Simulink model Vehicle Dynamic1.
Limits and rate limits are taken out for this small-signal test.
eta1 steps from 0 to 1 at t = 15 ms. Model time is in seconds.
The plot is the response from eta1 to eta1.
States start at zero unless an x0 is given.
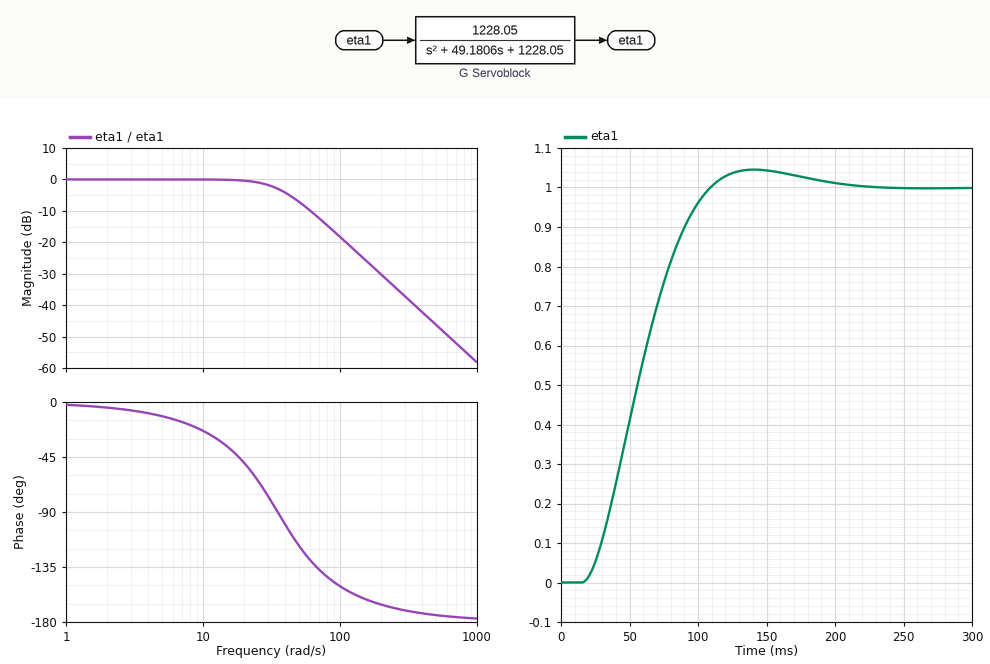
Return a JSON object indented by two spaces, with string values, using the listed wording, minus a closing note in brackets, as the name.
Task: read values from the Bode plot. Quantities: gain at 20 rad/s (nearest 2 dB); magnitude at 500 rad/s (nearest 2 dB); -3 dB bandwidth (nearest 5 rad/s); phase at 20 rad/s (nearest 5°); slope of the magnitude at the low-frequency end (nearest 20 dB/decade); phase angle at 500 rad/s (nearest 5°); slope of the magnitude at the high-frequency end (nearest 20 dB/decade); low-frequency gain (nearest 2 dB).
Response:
{
  "gain at 20 rad/s": "0 dB",
  "magnitude at 500 rad/s": "-46 dB",
  "-3 dB bandwidth": "35 rad/s",
  "phase at 20 rad/s": "-50°",
  "slope of the magnitude at the low-frequency end": "0 dB/decade",
  "phase angle at 500 rad/s": "-175°",
  "slope of the magnitude at the high-frequency end": "-40 dB/decade",
  "low-frequency gain": "0 dB"
}
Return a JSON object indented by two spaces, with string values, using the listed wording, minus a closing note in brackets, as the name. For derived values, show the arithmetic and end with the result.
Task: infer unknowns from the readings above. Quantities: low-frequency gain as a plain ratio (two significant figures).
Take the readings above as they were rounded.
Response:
{
  "low-frequency gain as a plain ratio": "10^(0 / 20) = 1.0"
}
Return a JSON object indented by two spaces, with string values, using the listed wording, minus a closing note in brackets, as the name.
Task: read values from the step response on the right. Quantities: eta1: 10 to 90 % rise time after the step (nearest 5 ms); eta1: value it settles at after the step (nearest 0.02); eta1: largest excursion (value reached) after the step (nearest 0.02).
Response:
{
  "eta1: 10 to 90 % rise time after the step": "60 ms",
  "eta1: value it settles at after the step": "1.00",
  "eta1: largest excursion (value reached) after the step": "1.04"
}
